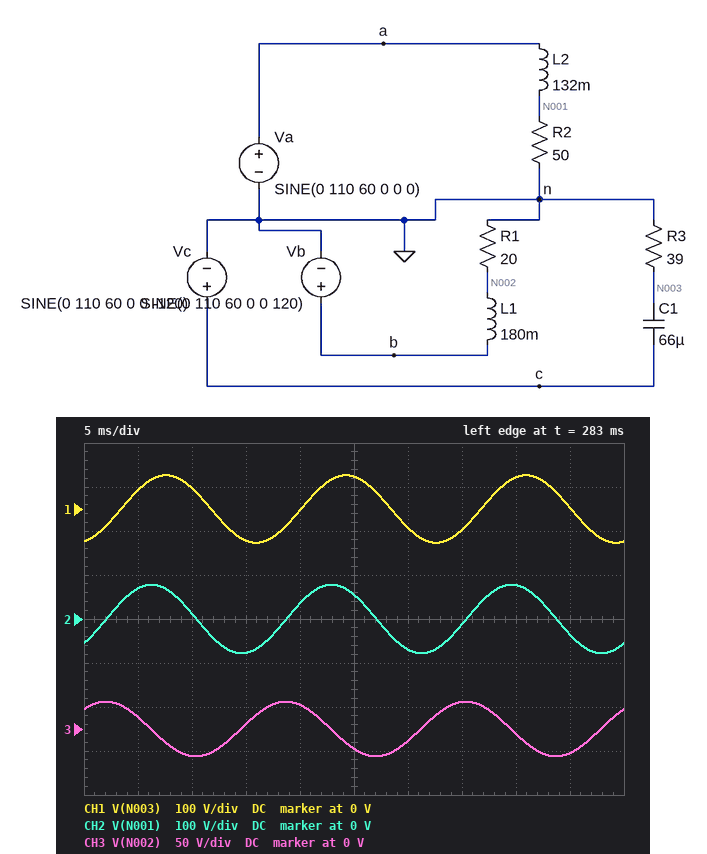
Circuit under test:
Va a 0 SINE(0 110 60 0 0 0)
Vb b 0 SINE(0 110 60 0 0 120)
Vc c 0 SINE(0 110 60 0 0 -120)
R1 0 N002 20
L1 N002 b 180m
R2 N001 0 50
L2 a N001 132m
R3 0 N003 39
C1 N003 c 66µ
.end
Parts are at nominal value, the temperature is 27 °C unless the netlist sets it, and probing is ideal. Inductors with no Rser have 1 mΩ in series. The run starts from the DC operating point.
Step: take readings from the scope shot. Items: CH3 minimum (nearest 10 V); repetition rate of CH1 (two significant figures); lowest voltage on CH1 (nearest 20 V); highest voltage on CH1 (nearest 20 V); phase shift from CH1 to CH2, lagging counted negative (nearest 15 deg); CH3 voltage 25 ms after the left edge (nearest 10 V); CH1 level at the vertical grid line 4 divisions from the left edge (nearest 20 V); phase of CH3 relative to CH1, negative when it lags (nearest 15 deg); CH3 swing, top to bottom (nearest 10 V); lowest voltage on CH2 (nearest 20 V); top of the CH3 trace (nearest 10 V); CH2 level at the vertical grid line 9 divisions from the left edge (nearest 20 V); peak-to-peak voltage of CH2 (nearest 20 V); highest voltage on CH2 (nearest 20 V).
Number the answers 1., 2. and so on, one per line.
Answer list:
1. -30 V
2. 60 Hz
3. -80 V
4. 80 V
5. 30 deg
6. -20 V
7. 0 V
8. 120 deg
9. 60 V
10. -80 V
11. 30 V
12. -40 V
13. 160 V
14. 80 V
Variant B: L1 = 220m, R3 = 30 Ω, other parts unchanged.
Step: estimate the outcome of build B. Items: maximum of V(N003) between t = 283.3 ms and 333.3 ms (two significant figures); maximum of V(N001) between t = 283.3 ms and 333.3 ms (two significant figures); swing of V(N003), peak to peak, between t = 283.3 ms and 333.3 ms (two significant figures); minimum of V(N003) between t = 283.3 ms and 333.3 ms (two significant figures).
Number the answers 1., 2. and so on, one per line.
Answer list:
1. 66 V
2. 78 V
3. 130 V
4. -66 V
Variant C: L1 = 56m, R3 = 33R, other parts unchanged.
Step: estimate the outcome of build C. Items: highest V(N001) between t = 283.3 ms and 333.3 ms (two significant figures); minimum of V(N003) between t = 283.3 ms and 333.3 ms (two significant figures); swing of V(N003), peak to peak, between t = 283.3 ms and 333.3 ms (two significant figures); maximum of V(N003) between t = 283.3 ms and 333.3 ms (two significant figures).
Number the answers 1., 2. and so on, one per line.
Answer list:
1. 78 V
2. -70 V
3. 140 V
4. 70 V
